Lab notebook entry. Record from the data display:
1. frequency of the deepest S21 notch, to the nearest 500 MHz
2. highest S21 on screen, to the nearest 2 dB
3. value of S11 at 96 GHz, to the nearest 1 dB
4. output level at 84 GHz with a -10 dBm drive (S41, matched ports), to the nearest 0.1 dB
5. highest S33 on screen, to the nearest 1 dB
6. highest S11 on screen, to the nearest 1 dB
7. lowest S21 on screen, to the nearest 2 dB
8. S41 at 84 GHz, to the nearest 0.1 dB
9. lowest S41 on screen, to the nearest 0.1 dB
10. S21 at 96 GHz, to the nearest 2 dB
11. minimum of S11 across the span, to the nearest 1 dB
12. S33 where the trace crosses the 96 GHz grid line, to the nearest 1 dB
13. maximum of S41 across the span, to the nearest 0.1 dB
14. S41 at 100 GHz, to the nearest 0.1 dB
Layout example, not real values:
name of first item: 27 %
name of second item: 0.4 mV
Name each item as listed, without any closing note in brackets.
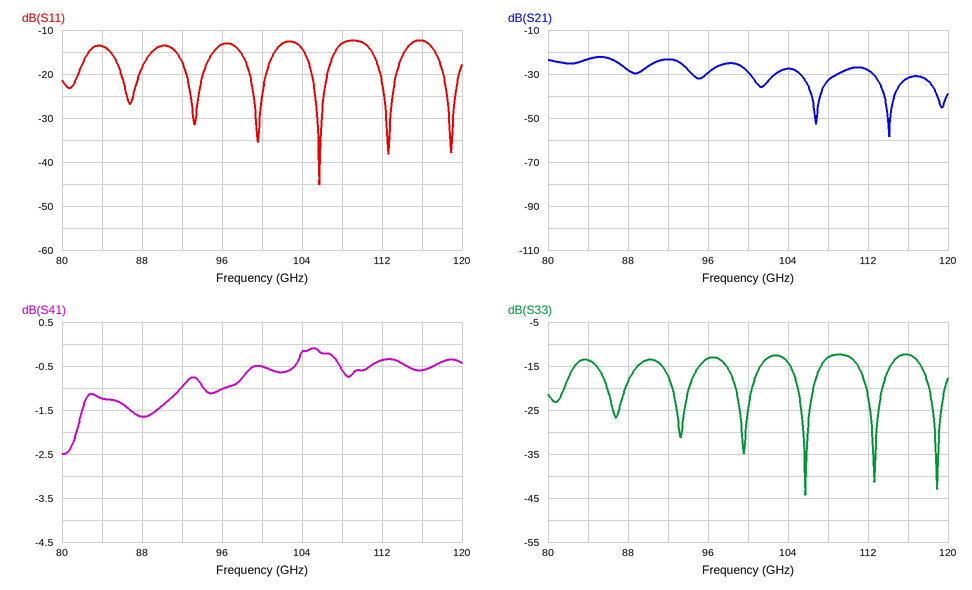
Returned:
frequency of the deepest S21 notch, to the nearest 500 MHz: 114.0 GHz
highest S21 on screen, to the nearest 2 dB: -22 dB
value of S11 at 96 GHz, to the nearest 1 dB: -13 dB
output level at 84 GHz with a -10 dBm drive (S41, matched ports), to the nearest 0.1 dB: -11.2 dBm
highest S33 on screen, to the nearest 1 dB: -12 dB
highest S11 on screen, to the nearest 1 dB: -12 dB
lowest S21 on screen, to the nearest 2 dB: -58 dB
S41 at 84 GHz, to the nearest 0.1 dB: -1.2 dB
lowest S41 on screen, to the nearest 0.1 dB: -2.5 dB
S21 at 96 GHz, to the nearest 2 dB: -30 dB
minimum of S11 across the span, to the nearest 1 dB: -45 dB
S33 where the trace crosses the 96 GHz grid line, to the nearest 1 dB: -13 dB
maximum of S41 across the span, to the nearest 0.1 dB: -0.1 dB
S41 at 100 GHz, to the nearest 0.1 dB: -0.5 dB
